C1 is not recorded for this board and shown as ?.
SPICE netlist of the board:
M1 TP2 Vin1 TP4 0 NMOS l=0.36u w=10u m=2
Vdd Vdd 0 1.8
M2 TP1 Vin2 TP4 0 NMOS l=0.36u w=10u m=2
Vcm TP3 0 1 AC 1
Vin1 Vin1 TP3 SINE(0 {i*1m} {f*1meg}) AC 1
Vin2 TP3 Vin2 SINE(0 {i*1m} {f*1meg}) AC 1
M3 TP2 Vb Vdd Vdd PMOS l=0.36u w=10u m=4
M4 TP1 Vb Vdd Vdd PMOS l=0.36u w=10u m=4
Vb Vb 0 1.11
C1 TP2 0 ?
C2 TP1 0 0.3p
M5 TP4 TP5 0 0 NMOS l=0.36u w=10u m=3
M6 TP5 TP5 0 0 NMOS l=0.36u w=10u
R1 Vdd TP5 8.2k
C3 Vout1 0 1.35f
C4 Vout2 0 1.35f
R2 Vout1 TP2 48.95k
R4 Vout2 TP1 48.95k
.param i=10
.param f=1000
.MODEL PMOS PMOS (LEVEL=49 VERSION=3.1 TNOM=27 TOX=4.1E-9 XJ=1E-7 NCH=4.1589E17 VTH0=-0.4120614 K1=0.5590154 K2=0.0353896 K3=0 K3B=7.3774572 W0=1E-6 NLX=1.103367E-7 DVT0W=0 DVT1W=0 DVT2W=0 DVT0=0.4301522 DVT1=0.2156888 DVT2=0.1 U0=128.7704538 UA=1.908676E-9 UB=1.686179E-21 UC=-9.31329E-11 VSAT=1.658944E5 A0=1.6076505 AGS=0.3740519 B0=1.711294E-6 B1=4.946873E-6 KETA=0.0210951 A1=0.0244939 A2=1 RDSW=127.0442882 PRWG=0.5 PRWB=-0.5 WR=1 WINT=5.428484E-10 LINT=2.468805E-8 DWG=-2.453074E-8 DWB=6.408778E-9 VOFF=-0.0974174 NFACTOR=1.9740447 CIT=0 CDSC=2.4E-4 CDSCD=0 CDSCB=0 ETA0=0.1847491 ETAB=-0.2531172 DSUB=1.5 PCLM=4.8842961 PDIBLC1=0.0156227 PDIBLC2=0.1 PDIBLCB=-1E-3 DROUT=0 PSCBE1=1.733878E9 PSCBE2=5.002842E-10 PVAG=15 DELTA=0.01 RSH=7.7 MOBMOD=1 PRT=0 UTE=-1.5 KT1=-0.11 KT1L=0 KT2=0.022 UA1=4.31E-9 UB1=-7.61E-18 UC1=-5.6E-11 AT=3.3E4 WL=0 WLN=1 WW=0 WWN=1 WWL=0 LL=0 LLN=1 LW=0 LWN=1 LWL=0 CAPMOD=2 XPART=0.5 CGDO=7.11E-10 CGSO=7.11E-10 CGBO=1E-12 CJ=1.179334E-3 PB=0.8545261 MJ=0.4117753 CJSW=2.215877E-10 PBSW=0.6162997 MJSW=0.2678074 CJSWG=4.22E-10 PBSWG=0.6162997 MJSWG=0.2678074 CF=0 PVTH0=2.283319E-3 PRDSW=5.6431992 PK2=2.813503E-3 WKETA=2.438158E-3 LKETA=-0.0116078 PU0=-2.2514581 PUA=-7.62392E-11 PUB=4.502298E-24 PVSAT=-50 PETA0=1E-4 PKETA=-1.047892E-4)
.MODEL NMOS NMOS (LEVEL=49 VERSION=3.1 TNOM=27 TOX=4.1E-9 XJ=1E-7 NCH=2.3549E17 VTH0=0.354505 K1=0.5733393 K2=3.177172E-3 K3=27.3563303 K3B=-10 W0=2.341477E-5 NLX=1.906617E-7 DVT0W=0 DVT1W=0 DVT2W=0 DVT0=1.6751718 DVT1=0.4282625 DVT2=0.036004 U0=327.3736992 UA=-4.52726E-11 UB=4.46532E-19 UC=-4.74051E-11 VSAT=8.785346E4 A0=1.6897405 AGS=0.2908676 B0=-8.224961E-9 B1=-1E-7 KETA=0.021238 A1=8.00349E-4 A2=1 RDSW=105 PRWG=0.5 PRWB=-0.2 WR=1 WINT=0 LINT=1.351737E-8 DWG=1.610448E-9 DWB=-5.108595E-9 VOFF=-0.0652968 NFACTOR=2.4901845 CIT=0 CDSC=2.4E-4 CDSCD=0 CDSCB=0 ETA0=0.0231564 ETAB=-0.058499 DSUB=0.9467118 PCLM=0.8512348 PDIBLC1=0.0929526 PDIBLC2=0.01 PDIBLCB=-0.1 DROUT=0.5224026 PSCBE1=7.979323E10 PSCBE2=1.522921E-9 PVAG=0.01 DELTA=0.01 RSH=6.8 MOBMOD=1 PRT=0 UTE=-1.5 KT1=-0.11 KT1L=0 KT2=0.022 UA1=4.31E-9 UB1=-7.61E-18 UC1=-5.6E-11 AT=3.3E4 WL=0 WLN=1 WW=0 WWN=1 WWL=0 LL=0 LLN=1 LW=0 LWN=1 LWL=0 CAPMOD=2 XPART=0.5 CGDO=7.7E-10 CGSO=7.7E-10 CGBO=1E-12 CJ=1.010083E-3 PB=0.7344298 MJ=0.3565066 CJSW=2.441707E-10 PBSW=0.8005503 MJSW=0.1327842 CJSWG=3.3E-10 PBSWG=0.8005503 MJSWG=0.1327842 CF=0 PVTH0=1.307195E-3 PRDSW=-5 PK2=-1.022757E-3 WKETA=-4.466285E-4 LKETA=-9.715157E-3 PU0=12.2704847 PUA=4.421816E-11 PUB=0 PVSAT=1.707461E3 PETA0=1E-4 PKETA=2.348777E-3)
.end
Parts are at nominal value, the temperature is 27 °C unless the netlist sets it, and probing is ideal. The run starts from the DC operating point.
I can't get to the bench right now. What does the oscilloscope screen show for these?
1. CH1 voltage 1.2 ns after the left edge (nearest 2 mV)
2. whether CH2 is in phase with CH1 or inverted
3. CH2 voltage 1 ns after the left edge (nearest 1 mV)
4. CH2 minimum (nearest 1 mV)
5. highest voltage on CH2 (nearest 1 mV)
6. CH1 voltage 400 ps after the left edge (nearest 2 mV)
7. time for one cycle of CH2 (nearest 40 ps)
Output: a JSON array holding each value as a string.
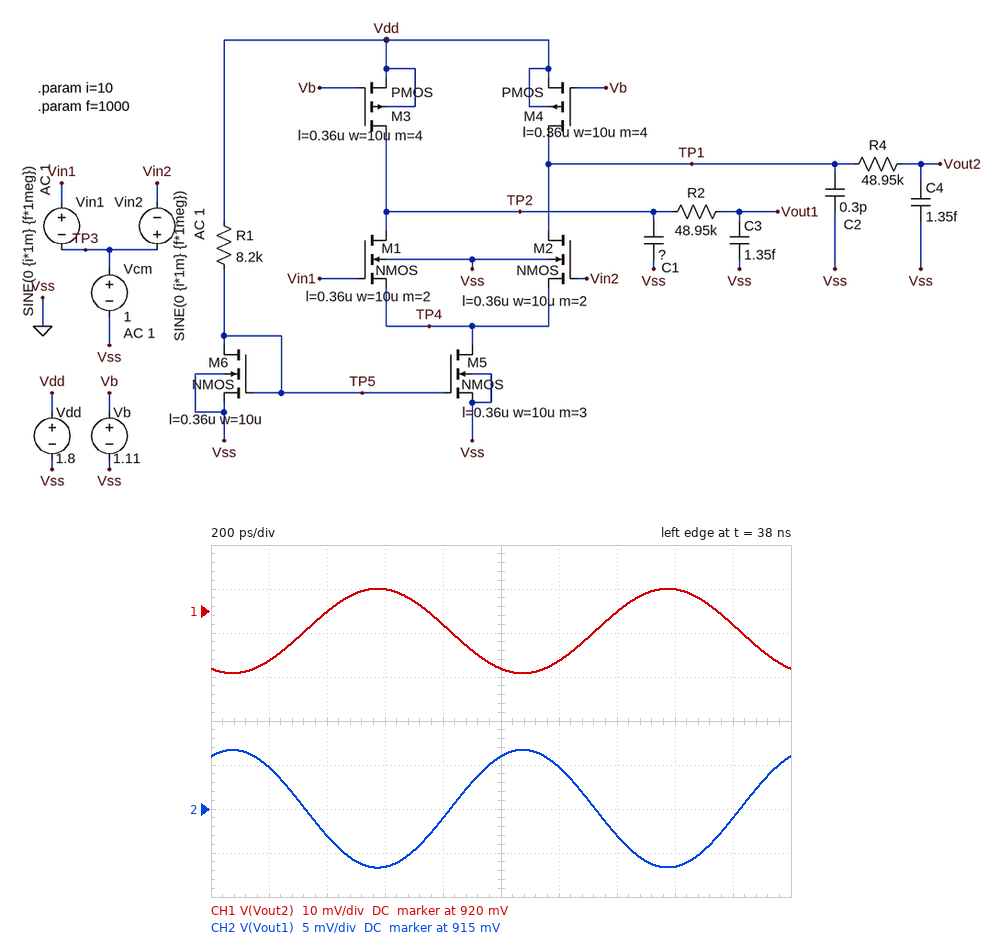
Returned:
["908 mV", "inverted", "921 mV", "908 mV", "922 mV", "920 mV", "1.00 ns"]
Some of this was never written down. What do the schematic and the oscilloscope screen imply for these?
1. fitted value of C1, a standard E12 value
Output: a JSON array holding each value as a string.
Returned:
["470 fF"]
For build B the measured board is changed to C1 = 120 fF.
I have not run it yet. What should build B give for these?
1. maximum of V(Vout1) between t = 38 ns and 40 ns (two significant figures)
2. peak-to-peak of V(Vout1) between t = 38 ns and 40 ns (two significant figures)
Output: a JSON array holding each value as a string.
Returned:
["940 mV", "42 mV"]
